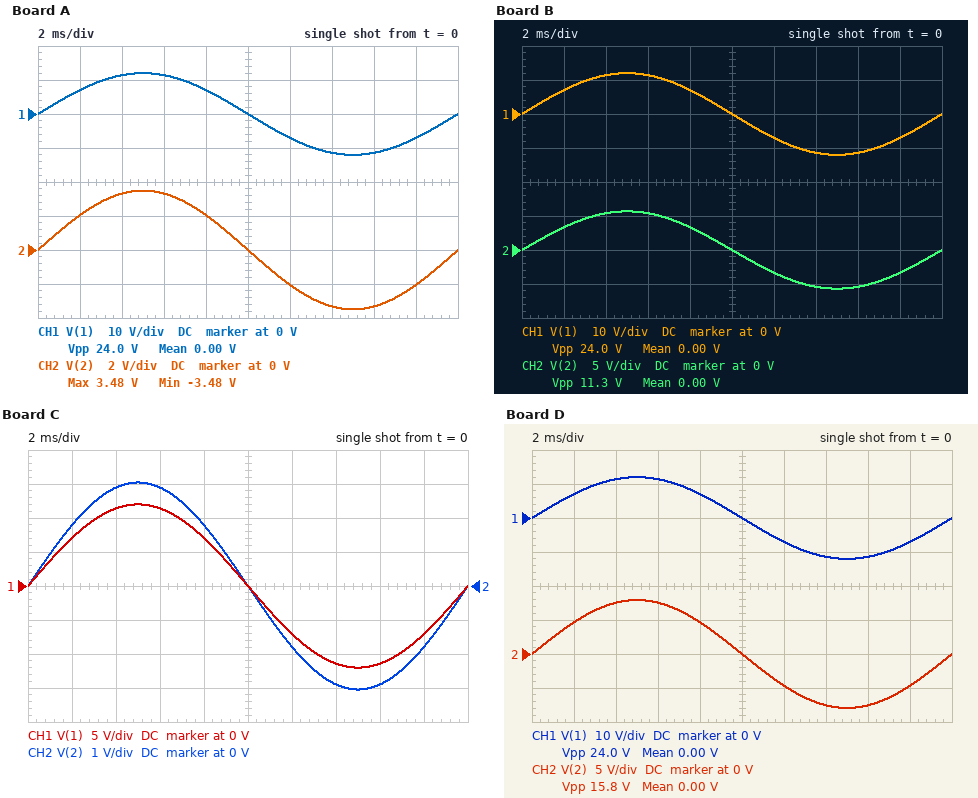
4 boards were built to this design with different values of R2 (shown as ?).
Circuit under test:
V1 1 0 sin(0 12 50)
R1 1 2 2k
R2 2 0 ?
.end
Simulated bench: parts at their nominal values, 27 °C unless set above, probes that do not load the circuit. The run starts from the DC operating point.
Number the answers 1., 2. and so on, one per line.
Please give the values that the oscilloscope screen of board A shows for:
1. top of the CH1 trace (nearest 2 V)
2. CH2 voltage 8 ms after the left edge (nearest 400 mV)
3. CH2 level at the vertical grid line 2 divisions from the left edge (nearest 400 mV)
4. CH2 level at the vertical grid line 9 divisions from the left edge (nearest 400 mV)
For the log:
1. 12 V
2. 2.0 V
3. 3.2 V
4. -2.0 V
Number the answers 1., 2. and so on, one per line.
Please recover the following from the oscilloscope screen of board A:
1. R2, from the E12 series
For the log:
1. 820 Ω
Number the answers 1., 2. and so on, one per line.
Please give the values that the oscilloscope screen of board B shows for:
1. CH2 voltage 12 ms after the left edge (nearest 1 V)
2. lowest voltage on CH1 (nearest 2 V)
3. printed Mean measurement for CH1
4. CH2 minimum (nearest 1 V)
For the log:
1. -3 V
2. -12 V
3. 0.00 V
4. -6 V
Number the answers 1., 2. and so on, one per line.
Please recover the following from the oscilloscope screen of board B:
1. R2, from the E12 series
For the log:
1. 1.8 kΩ
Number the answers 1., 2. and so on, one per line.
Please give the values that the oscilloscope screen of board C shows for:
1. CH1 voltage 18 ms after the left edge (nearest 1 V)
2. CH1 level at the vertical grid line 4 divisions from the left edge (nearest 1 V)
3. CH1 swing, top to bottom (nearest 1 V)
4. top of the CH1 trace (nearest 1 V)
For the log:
1. -7 V
2. 7 V
3. 24 V
4. 12 V
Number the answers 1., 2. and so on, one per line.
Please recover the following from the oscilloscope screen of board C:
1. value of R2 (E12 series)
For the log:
1. 680 Ω
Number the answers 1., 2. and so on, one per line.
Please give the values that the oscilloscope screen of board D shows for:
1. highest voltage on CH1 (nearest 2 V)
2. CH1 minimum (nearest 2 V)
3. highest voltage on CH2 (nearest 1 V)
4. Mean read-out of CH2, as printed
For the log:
1. 12 V
2. -12 V
3. 8 V
4. 0.00 V
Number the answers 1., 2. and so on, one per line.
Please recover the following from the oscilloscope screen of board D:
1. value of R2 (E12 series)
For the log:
1. 3.9 kΩ
